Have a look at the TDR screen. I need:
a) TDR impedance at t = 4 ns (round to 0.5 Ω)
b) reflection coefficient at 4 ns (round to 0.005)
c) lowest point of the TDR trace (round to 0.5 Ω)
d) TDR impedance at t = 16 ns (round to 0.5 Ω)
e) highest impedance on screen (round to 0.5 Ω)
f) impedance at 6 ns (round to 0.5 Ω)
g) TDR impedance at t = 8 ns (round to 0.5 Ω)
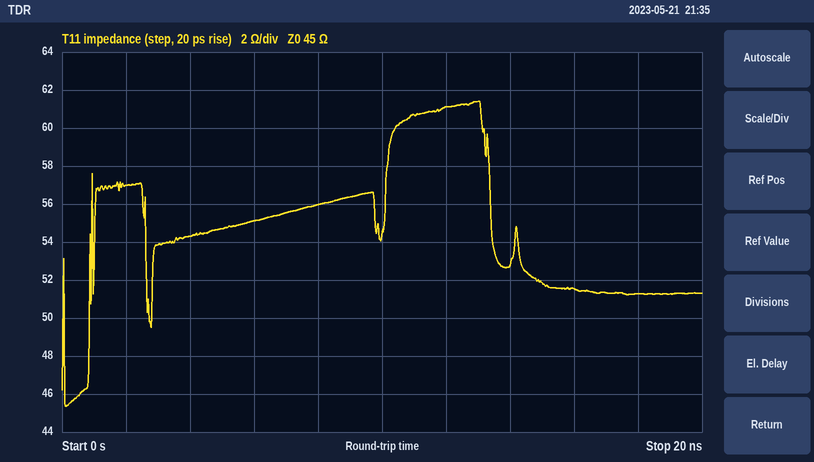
54.5 Ω
+0.095
45.5 Ω
51.5 Ω
61.5 Ω
55.0 Ω
56.0 Ω
